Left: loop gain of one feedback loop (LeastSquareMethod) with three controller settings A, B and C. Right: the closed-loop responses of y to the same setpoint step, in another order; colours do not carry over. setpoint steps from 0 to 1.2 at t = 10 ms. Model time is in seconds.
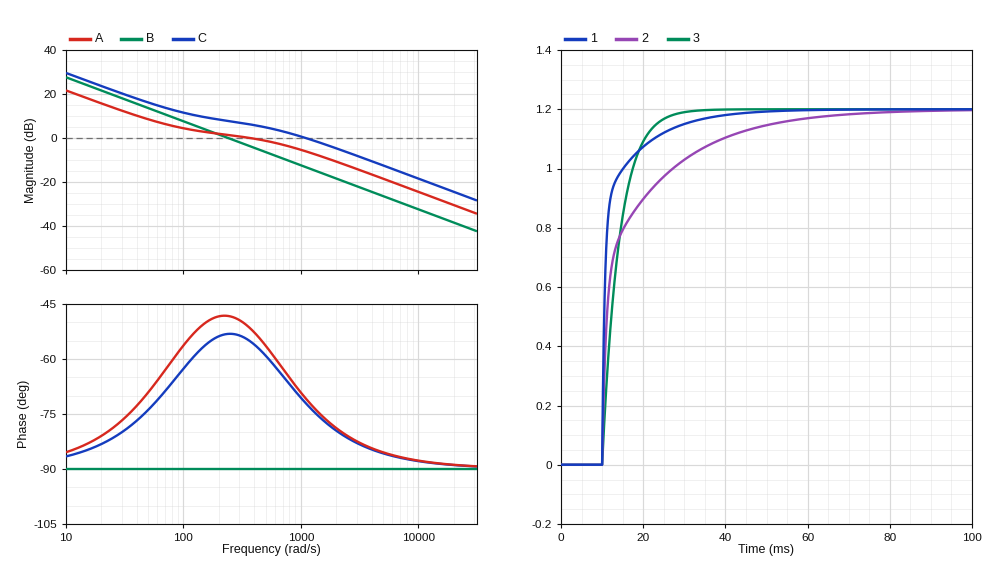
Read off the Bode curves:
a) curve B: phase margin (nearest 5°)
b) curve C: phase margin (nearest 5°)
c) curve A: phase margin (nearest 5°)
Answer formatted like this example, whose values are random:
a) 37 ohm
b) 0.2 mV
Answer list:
a) 90°
b) 110°
c) 130°
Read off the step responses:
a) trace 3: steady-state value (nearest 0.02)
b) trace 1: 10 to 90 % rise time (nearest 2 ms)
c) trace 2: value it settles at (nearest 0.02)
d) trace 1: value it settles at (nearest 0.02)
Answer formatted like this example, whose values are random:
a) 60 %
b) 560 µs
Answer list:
a) 1.20
b) 10 ms
c) 1.20
d) 1.20
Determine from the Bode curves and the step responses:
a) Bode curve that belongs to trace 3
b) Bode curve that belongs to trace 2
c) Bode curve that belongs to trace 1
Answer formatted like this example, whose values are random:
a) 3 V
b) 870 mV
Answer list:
a) B
b) A
c) C
